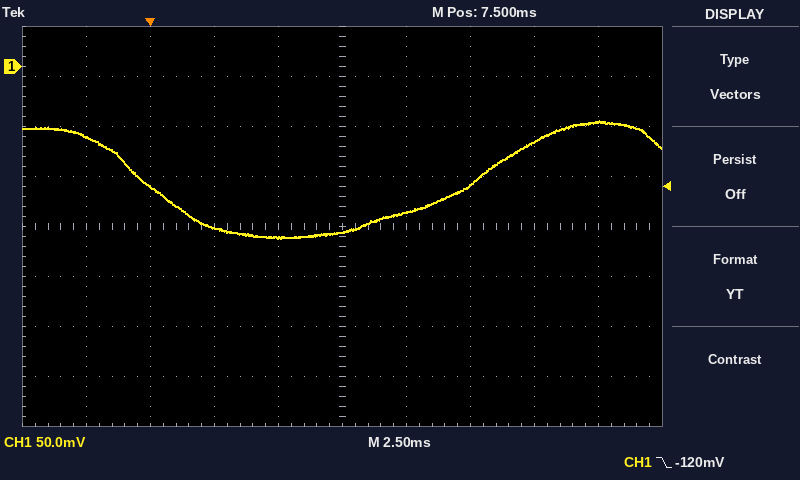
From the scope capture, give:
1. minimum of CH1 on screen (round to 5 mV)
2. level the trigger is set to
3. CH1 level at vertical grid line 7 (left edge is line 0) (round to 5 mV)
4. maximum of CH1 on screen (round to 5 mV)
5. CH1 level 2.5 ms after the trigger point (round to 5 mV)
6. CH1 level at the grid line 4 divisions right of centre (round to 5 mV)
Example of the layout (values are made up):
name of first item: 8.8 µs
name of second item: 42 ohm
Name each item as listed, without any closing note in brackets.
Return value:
minimum of CH1 on screen: -170 mV
level the trigger is set to: -120 mV
CH1 level at vertical grid line 7 (left edge is line 0): -120 mV
maximum of CH1 on screen: -55 mV
CH1 level 2.5 ms after the trigger point: -160 mV
CH1 level at the grid line 4 divisions right of centre: -55 mV
